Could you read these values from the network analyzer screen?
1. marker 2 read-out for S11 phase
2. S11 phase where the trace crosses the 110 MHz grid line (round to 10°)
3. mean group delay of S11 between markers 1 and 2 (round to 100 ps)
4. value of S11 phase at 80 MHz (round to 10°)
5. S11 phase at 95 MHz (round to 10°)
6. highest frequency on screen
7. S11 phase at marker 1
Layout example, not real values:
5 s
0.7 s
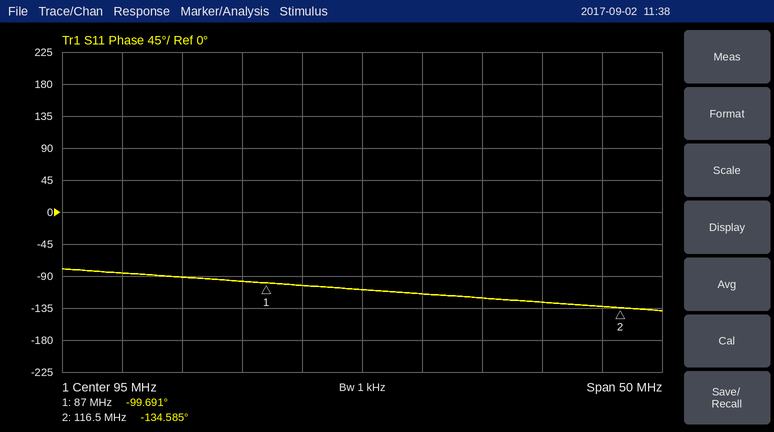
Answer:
-134.585°
-130°
3.3 ns
-90°
-110°
120 MHz
-99.691°
